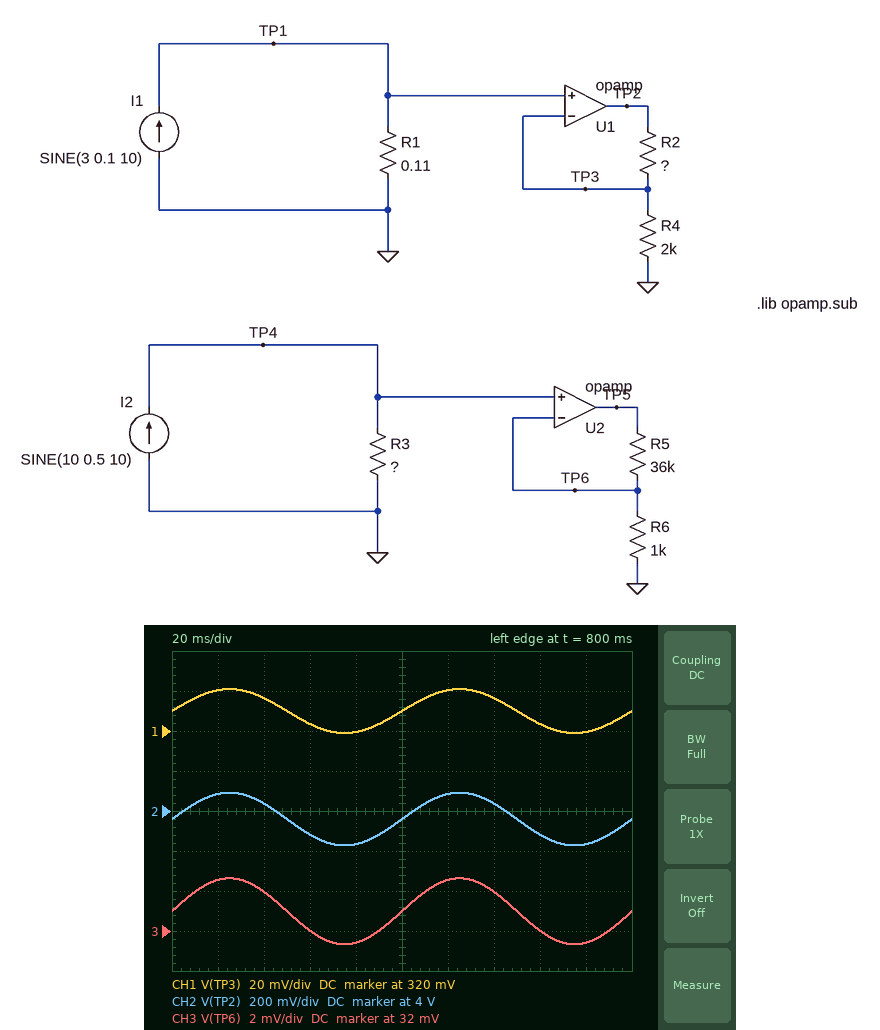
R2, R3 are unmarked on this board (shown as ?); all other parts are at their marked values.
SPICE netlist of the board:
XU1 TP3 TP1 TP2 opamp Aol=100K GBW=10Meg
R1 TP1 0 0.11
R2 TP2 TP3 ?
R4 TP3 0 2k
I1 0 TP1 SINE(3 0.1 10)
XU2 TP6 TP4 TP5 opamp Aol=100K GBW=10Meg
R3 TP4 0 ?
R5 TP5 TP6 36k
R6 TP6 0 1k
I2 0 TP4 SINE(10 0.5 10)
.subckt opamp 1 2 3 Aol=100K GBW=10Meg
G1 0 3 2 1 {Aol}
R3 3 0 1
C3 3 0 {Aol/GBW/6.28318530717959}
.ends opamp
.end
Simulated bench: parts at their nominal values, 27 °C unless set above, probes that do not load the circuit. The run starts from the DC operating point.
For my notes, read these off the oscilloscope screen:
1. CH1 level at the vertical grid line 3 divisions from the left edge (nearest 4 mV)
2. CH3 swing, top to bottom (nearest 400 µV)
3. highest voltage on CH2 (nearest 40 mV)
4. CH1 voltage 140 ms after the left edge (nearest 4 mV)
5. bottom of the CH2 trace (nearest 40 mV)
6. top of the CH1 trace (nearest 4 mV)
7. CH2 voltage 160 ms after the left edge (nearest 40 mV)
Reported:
324 mV
3.2 mV
4.08 V
336 mV
3.84 V
340 mV
3.88 V
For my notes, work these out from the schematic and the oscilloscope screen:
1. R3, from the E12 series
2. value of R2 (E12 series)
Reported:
3.3 mΩ
22 kΩ
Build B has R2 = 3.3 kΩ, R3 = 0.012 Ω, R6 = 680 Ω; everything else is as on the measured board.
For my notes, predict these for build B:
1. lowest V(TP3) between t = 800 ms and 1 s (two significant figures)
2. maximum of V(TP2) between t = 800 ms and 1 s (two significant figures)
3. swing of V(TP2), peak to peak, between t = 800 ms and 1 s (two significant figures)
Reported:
320 mV
900 mV
58 mV
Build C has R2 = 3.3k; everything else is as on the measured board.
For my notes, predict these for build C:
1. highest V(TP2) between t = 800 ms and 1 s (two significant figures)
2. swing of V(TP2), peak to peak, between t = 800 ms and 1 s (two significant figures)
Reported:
900 mV
58 mV
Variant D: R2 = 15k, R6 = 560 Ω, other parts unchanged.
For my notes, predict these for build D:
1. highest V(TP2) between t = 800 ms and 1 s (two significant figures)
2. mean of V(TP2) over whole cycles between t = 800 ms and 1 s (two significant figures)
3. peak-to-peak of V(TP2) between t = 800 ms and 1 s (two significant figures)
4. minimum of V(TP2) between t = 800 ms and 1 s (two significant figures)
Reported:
2.9 V
2.8 V
190 mV
2.7 V
